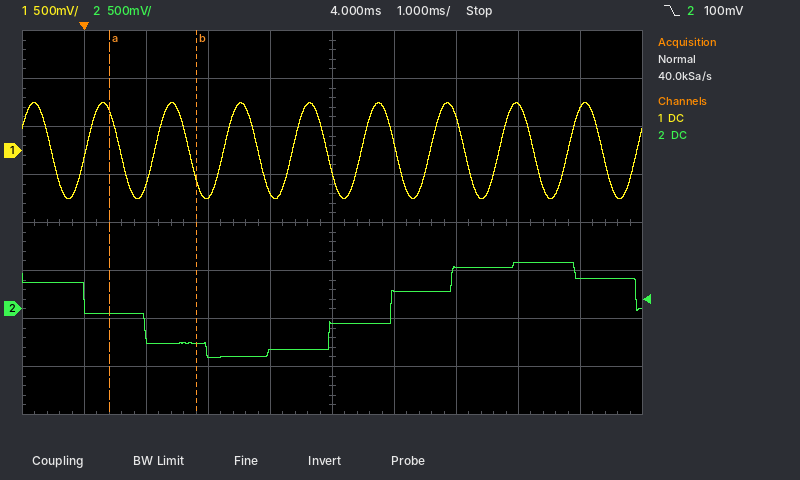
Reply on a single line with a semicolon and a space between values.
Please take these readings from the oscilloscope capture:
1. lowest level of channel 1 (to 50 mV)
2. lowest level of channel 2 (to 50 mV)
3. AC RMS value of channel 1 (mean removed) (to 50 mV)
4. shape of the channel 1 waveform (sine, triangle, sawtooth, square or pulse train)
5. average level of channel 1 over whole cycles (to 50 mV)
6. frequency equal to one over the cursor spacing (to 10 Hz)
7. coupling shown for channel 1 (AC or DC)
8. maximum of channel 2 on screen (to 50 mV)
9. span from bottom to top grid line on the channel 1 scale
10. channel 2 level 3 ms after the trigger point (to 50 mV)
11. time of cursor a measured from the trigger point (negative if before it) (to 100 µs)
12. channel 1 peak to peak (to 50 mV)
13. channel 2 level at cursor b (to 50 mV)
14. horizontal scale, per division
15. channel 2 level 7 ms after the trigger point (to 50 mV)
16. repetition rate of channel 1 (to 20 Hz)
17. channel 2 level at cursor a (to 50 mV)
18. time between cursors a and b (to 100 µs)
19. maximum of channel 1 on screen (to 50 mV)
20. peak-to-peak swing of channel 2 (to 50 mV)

-500 mV; -500 mV; 350 mV; sine; 0 mV; 710 Hz; DC; 500 mV; 4 V; -450 mV; +400 µs; 1.00 V; -350 mV; 1 ms; 500 mV; 900 Hz; -50 mV; 1.4 ms; 500 mV; 1.00 V
